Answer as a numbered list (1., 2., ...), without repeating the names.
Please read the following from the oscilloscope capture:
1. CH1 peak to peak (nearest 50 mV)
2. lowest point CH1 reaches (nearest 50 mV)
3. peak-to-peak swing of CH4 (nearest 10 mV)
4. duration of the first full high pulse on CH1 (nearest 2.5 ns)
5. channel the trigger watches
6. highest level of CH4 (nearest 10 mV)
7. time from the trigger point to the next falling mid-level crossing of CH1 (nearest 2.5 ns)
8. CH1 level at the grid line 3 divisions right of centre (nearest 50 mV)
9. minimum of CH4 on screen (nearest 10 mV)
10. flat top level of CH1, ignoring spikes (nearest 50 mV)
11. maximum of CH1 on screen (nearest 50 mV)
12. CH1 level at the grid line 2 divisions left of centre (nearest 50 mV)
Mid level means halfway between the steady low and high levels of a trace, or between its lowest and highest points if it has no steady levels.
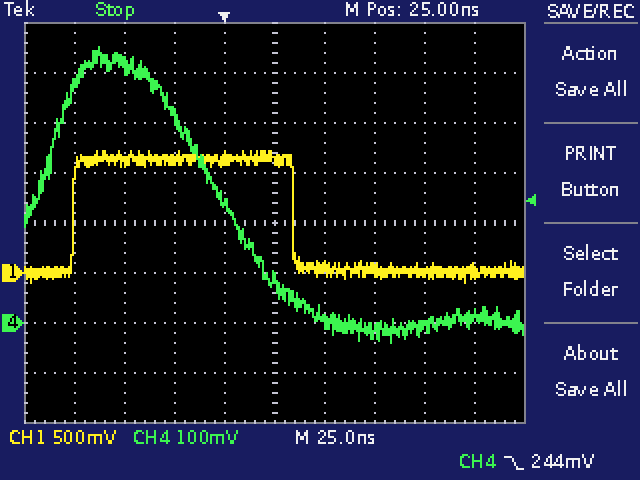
1. 1.30 V
2. -100 mV
3. 590 mV
4. 110.0 ns
5. CH4
6. 550 mV
7. 35.0 ns
8. 0 mV
9. -40 mV
10. 1.15 V
11. 1.20 V
12. 1.15 V
